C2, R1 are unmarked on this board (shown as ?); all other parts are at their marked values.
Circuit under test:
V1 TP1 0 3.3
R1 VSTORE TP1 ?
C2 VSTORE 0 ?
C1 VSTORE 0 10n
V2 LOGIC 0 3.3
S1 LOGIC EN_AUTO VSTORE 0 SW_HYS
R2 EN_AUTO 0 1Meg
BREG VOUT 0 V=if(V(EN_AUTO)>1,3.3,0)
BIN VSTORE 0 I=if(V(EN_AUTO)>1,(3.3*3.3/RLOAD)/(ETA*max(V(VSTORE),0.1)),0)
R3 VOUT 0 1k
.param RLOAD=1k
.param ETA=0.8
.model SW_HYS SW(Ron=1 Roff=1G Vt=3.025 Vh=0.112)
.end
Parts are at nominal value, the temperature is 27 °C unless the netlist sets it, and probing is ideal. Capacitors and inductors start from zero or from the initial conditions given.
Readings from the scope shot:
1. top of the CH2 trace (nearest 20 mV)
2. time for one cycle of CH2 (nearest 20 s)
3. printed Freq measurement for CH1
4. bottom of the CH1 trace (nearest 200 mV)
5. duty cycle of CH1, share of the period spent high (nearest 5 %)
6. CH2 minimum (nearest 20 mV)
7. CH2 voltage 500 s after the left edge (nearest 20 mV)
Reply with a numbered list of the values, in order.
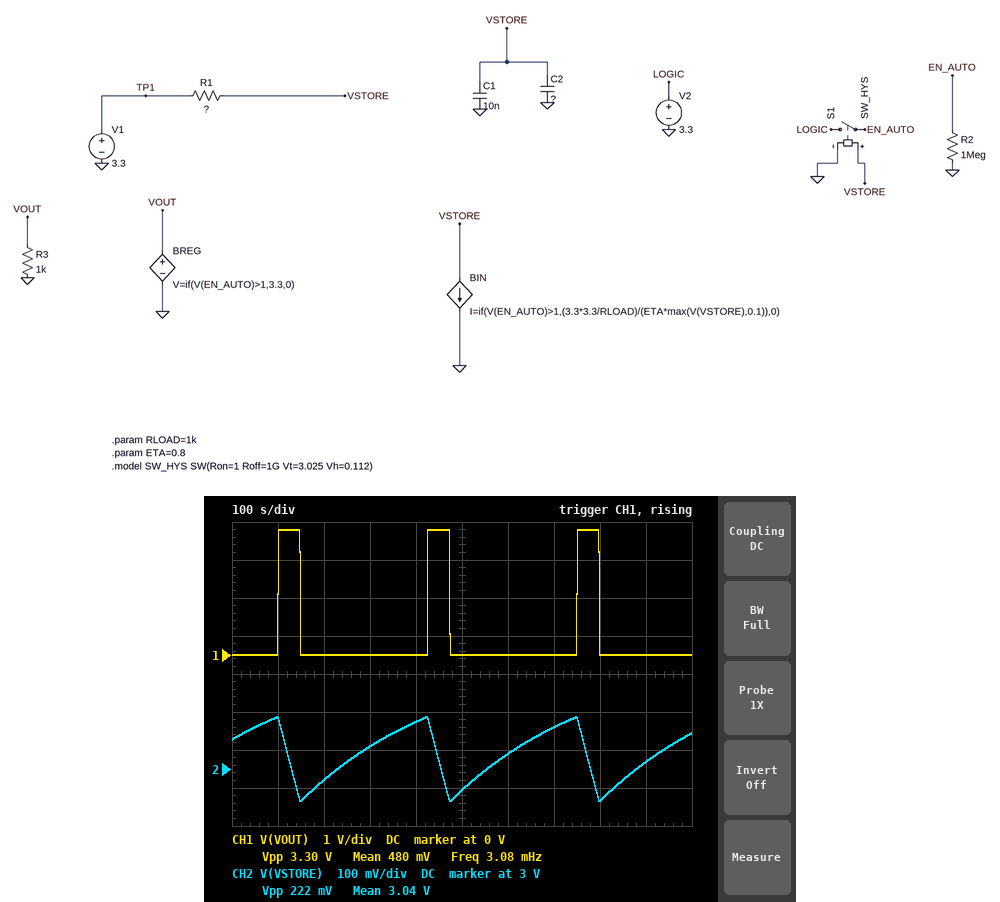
1. 3.14 V
2. 320 s
3. 3.08 mHz
4. 0 V
5. 15 %
6. 2.92 V
7. 2.94 V
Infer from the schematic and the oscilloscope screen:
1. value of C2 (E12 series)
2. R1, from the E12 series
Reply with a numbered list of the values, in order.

1. 820 mF
2. 390 Ω
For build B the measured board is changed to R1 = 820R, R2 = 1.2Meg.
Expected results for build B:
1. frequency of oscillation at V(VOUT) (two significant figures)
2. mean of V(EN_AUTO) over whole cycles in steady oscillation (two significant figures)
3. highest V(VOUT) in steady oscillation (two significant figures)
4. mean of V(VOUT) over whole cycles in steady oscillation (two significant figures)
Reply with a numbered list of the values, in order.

1. 1.6 mHz
2. 240 mV
3. 3.3 V
4. 230 mV
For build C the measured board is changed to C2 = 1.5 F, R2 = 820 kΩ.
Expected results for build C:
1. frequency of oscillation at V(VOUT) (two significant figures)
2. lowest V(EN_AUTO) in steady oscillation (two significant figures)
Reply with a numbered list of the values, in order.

1. 1.7 mHz
2. 2.7 mV
